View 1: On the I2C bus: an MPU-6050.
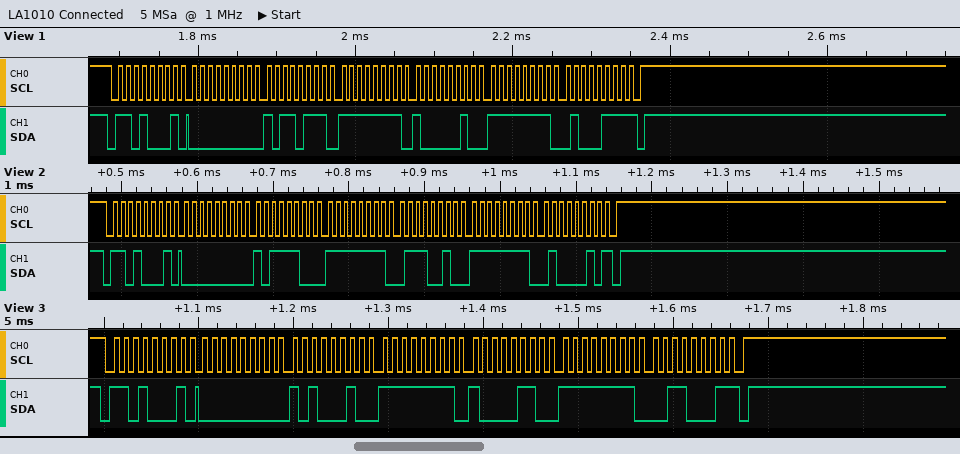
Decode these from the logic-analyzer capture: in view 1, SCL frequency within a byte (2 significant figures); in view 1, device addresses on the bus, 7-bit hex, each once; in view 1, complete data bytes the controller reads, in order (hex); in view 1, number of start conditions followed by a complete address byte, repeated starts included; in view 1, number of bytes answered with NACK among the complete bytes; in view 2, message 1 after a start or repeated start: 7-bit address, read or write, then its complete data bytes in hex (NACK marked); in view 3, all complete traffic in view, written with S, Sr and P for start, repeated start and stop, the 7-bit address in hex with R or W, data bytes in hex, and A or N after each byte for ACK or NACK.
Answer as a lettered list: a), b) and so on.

a) 100 kHz
b) 0x68
c) 00 B7 FF 82 FF 47
d) 1
e) 1
f) 0x68 read: 00 BC FF 72 FF 42 NACK
g) S 68R A 00 A A2 A FF A 86 A FF A 31 N P
